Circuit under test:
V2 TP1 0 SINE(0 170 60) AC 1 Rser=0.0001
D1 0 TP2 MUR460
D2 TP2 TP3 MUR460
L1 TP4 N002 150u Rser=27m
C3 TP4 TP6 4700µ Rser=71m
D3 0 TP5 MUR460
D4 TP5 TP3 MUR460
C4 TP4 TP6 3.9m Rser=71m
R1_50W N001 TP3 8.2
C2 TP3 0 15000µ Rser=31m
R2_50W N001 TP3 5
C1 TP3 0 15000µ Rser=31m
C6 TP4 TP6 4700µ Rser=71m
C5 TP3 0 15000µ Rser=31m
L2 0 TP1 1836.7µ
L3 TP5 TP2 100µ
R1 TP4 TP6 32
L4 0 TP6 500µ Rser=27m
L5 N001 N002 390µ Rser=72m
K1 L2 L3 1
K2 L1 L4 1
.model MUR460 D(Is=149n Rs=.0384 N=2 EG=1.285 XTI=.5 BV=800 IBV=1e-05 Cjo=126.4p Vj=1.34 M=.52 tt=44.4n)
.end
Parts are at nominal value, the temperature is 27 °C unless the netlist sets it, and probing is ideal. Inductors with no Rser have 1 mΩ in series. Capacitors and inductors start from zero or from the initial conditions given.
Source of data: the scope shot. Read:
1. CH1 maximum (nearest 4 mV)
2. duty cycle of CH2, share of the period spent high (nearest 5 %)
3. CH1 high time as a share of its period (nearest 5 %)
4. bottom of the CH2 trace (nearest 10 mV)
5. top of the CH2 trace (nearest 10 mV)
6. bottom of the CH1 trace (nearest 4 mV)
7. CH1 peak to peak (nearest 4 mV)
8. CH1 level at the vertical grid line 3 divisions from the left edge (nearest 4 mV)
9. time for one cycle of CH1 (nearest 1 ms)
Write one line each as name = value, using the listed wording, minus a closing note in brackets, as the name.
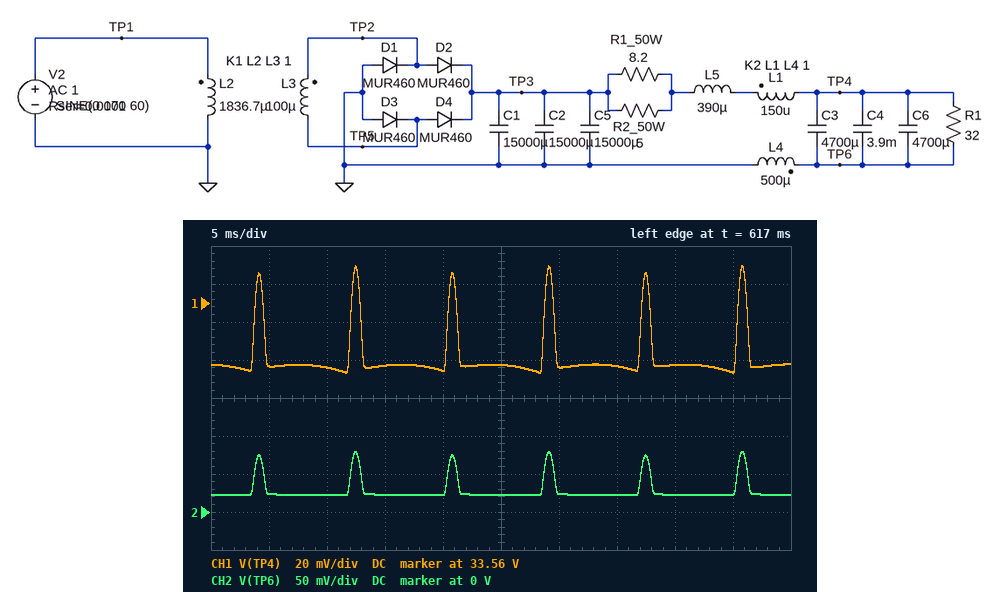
CH1 maximum = 33.580 V
duty cycle of CH2, share of the period spent high = 10 %
CH1 high time as a share of its period = 10 %
bottom of the CH2 trace = 20 mV
top of the CH2 trace = 80 mV
bottom of the CH1 trace = 33.524 V
CH1 peak to peak = 56 mV
CH1 level at the vertical grid line 3 divisions from the left edge = 33.528 V
time for one cycle of CH1 = 8 ms
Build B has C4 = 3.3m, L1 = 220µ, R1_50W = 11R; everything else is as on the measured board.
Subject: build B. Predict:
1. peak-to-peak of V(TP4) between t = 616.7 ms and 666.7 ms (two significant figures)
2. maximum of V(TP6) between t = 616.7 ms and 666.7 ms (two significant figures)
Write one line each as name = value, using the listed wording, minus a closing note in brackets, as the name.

peak-to-peak of V(TP4) between t = 616.7 ms and 666.7 ms = 54 mV
maximum of V(TP6) between t = 616.7 ms and 666.7 ms = 77 mV
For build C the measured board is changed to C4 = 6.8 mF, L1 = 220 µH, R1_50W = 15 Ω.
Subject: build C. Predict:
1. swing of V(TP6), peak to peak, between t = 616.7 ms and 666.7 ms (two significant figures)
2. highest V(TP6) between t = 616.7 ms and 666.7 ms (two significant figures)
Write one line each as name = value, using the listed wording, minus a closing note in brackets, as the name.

swing of V(TP6), peak to peak, between t = 616.7 ms and 666.7 ms = 52 mV
highest V(TP6) between t = 616.7 ms and 666.7 ms = 74 mV
